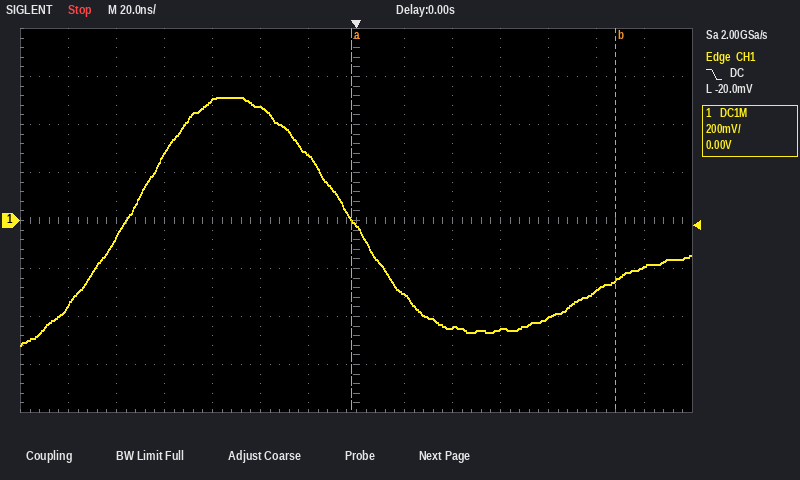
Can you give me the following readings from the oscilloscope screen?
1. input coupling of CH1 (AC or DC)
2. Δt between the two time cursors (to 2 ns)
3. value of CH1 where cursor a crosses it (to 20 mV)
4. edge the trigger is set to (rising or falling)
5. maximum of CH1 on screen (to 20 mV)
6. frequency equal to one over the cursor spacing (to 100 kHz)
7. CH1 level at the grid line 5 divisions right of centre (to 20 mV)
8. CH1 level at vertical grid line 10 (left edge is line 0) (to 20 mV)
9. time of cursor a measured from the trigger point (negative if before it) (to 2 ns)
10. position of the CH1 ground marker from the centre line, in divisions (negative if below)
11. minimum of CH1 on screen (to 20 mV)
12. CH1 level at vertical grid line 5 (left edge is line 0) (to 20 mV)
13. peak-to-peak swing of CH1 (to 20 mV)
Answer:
DC
110 ns
0 mV
falling
520 mV
9.1 MHz
-300 mV
-460 mV
-2 ns
0.0 div
-520 mV
480 mV
1.04 V
